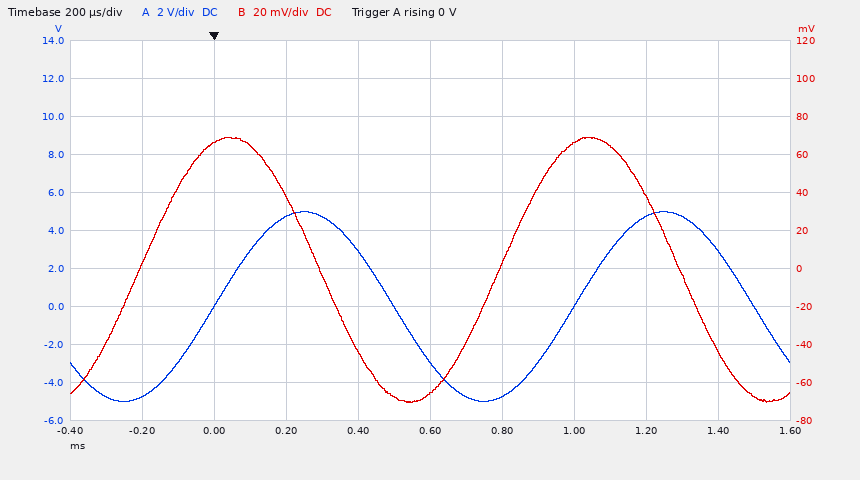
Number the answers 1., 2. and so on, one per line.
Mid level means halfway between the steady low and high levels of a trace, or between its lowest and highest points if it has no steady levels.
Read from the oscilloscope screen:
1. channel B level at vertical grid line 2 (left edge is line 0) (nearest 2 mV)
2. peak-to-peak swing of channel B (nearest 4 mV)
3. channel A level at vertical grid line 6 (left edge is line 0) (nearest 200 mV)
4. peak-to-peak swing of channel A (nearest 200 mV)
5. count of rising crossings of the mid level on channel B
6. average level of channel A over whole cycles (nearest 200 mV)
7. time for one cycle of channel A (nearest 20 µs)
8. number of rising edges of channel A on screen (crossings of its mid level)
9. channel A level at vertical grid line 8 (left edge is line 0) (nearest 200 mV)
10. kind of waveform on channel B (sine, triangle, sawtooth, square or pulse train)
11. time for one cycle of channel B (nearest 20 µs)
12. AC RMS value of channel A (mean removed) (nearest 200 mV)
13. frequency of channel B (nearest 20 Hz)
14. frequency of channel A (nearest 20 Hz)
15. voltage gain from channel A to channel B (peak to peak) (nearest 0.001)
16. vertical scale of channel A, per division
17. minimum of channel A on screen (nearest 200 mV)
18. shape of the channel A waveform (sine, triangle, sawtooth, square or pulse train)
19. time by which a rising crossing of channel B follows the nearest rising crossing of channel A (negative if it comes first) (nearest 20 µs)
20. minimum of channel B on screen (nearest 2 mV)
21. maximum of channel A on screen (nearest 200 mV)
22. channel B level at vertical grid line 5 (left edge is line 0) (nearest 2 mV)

1. 66 mV
2. 140 mV
3. -4.8 V
4. 10.0 V
5. 2
6. 0.0 V
7. 1.00 ms
8. 2
9. 4.8 V
10. sine
11. 1.00 ms
12. 3.6 V
13. 1.00 kHz
14. 1.00 kHz
15. 0.014
16. 2 V
17. -5.0 V
18. sine
19. -200 µs
20. -70 mV
21. 5.0 V
22. -66 mV
